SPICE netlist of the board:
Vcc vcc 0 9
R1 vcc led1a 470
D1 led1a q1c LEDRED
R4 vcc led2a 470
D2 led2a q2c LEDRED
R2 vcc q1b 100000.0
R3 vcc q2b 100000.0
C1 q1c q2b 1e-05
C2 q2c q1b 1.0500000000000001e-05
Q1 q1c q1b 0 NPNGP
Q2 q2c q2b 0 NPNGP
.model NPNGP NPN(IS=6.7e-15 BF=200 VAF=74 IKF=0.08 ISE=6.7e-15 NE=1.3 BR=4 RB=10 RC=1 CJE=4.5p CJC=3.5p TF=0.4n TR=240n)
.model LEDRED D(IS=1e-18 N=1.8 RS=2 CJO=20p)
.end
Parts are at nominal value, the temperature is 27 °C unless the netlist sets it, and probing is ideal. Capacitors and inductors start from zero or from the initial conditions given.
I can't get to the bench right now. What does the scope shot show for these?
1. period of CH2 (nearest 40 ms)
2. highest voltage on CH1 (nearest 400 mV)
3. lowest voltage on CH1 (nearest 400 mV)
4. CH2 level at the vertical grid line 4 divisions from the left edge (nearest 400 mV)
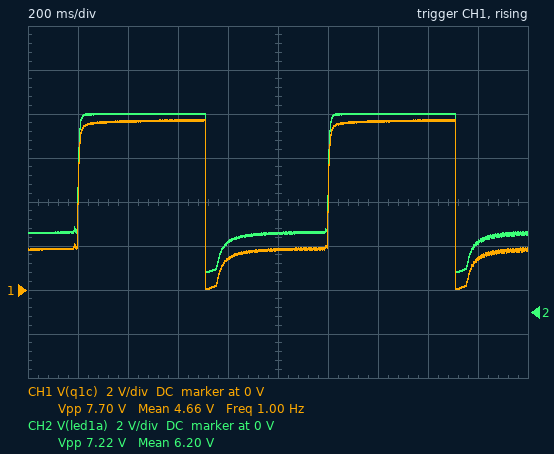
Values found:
1.00 s
7.6 V
0 V
3.2 V
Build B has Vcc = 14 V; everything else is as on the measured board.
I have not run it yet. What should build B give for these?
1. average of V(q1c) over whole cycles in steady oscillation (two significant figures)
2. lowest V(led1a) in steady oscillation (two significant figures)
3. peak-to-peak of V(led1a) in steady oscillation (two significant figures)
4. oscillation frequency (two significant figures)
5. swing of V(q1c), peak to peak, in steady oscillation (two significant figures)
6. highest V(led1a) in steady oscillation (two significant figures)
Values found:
8.1 V
1.9 V
12 V
1.0 Hz
13 V
14 V
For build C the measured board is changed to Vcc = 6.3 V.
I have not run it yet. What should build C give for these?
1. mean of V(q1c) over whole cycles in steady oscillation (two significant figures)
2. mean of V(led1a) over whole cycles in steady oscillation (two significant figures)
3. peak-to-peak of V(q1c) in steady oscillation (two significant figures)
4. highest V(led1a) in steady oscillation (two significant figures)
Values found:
2.9 V
4.4 V
5.0 V
6.3 V
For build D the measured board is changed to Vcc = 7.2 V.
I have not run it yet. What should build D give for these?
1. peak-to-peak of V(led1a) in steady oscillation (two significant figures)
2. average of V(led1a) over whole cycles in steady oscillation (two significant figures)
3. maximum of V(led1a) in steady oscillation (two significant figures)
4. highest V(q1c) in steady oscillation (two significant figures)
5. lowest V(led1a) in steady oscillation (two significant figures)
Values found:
5.4 V
5.0 V
7.2 V
5.9 V
1.8 V
